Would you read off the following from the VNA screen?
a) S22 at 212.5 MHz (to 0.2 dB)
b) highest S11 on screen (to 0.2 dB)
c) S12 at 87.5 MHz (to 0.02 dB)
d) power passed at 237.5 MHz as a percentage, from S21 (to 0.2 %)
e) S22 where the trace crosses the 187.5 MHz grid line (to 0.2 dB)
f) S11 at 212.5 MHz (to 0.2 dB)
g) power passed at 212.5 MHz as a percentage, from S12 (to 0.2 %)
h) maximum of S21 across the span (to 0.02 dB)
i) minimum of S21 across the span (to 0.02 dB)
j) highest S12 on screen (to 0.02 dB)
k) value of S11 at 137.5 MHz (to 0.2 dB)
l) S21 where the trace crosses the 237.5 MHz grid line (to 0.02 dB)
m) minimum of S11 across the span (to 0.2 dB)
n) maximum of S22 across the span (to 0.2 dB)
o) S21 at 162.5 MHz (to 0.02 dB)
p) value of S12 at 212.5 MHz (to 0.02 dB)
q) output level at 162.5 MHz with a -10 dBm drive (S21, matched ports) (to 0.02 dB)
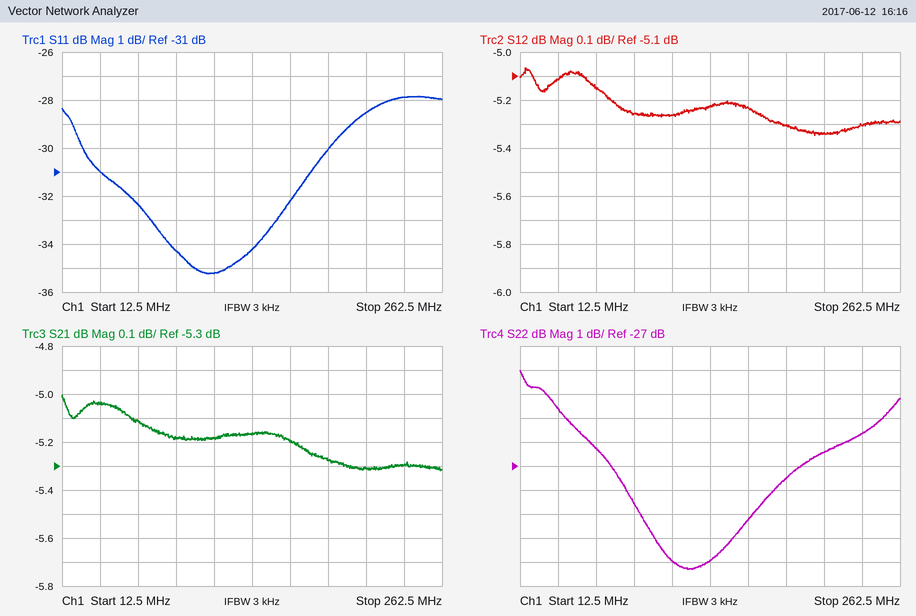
-26.4 dB
-27.8 dB
-5.26 dB
29.6 %
-27.6 dB
-28.6 dB
29.2 %
-5.00 dB
-5.32 dB
-5.06 dB
-34.2 dB
-5.30 dB
-35.2 dB
-23.0 dB
-5.20 dB
-5.34 dB
-15.20 dBm
